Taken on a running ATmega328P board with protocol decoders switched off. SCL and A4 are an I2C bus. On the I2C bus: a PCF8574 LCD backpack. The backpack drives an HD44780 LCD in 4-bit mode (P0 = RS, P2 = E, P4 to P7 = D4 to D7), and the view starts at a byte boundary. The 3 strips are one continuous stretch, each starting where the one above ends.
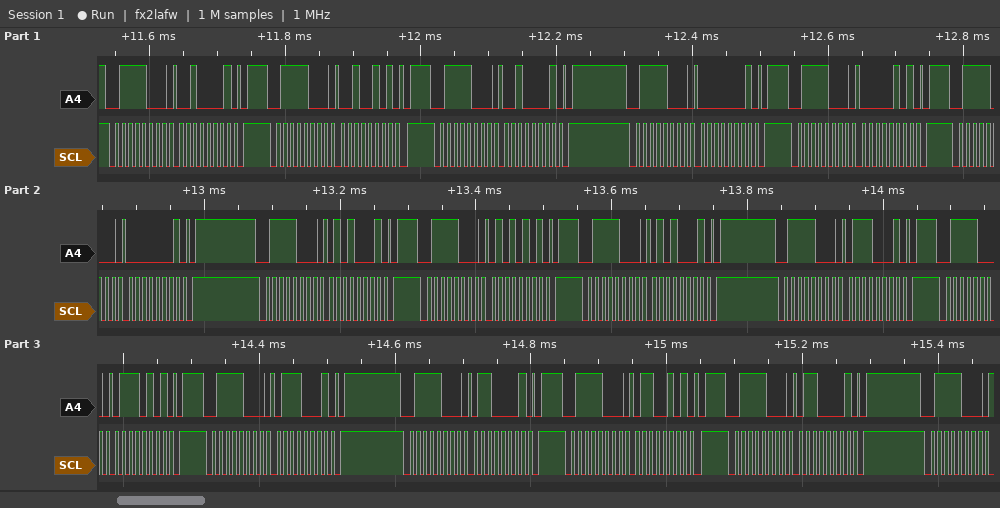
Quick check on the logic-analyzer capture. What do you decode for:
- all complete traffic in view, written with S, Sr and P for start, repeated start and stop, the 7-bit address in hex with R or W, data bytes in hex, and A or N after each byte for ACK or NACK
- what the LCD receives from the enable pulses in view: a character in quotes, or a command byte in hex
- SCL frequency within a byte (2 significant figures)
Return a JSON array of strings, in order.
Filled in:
["S 3CW A 21 A P S 3CW A 25 A P S 3CW A 21 A P S 3CW A 01 A P S 3CW A 05 A P S 3CW A 01 A P S 3CW A 51 A P S 3CW A 55 A P S 3CW A 51 A P S 3CW A 71 A P S 3CW A 75 A P S 3CW A 71 A P S 3CW A 61 A P S 3CW A 65 A P S 3CW A 61 A P S 3CW A", "' ' 'W'", "100 kHz"]
